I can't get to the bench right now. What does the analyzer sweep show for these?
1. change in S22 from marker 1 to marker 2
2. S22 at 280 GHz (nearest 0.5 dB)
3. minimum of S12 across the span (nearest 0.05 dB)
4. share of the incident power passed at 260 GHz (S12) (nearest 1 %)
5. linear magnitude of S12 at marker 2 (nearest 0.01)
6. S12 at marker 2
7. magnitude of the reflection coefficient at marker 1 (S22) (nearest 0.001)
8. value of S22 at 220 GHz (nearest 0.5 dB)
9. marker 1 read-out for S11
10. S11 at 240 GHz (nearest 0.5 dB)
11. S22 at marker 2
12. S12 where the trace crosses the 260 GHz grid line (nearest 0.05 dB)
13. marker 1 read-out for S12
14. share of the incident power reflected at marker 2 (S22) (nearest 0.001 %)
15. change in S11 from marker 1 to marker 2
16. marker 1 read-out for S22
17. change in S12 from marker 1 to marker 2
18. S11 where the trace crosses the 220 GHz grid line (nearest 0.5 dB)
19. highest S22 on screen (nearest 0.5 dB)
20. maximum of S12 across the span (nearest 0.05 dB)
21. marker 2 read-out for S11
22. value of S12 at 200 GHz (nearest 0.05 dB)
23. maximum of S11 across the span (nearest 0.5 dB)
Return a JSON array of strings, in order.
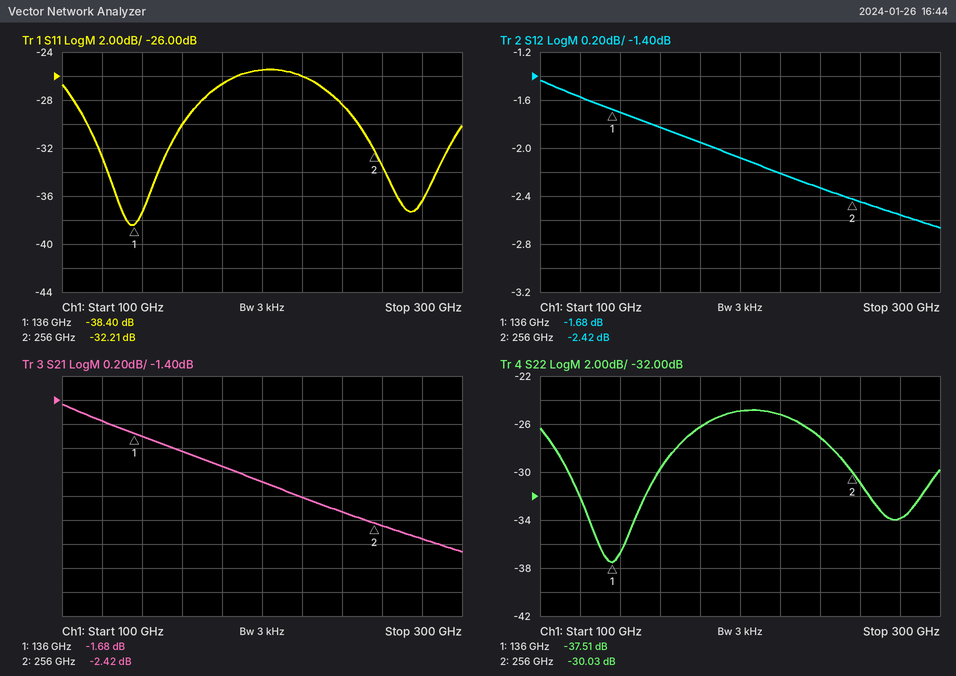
["7.48 dB", "-34.0 dB", "-2.65 dB", "57 %", "0.76", "-2.42 dB", "0.013", "-25.0 dB", "-38.40 dB", "-28.5 dB", "-30.03 dB", "-2.45 dB", "-1.68 dB", "0.099 %", "6.19 dB", "-37.51 dB", "-0.74 dB", "-26.0 dB", "-25.0 dB", "-1.45 dB", "-32.21 dB", "-2.10 dB", "-25.5 dB"]
